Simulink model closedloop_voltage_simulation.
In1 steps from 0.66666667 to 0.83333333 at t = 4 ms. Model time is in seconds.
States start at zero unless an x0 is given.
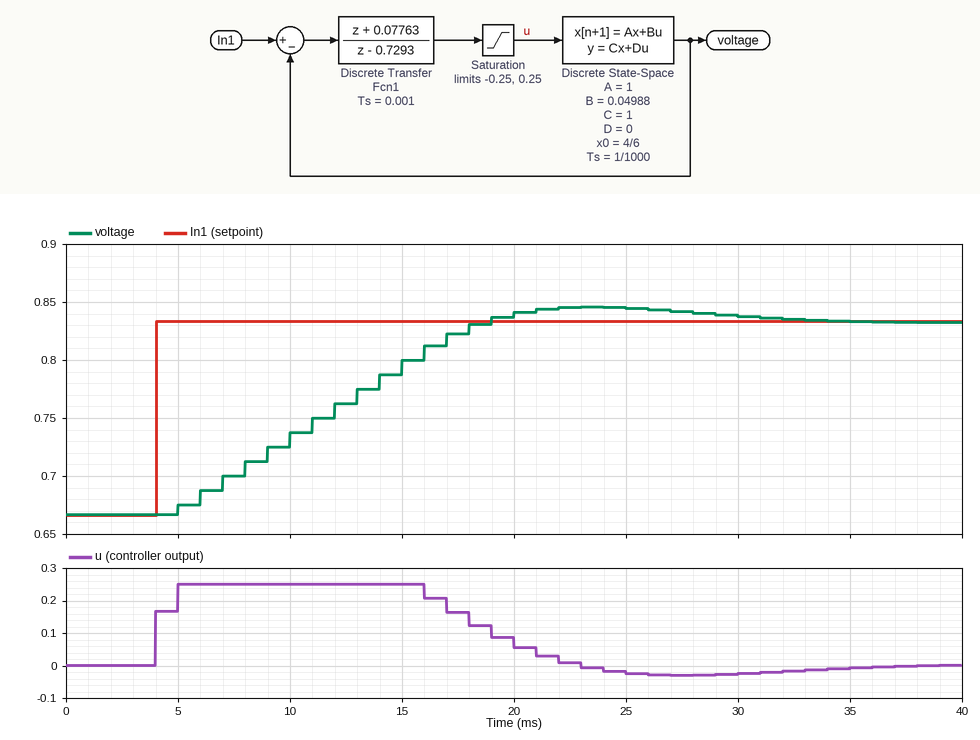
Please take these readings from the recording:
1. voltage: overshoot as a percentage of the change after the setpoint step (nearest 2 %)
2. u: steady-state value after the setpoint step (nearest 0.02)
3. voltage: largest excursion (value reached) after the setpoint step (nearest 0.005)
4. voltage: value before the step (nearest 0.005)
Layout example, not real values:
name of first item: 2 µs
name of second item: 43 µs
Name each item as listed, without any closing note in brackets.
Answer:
voltage: overshoot as a percentage of the change after the setpoint step: 8 %
u: steady-state value after the setpoint step: 0.00
voltage: largest excursion (value reached) after the setpoint step: 0.845
voltage: value before the step: 0.665
